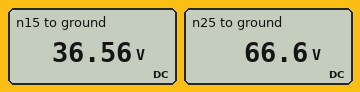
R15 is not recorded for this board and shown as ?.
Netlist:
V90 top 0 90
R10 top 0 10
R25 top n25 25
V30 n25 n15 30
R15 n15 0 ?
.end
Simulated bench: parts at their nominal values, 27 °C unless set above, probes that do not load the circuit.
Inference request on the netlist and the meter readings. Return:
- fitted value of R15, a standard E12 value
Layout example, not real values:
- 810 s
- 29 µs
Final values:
- 39 Ω
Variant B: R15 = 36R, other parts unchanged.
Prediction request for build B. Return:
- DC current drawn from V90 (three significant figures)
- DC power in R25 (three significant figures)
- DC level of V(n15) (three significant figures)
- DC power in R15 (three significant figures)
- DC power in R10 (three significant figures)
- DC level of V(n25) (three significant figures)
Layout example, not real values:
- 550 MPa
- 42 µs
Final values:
- 9.98 A
- 24.2 W
- 35.4 V
- 34.8 W
- 810 W
- 65.4 V
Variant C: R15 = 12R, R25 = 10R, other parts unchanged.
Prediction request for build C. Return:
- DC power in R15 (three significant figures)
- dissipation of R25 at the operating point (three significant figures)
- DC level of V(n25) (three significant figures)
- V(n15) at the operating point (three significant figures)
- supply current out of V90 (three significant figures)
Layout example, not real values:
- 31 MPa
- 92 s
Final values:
- 89.3 W
- 74.4 W
- 62.7 V
- 32.7 V
- 11.7 A
